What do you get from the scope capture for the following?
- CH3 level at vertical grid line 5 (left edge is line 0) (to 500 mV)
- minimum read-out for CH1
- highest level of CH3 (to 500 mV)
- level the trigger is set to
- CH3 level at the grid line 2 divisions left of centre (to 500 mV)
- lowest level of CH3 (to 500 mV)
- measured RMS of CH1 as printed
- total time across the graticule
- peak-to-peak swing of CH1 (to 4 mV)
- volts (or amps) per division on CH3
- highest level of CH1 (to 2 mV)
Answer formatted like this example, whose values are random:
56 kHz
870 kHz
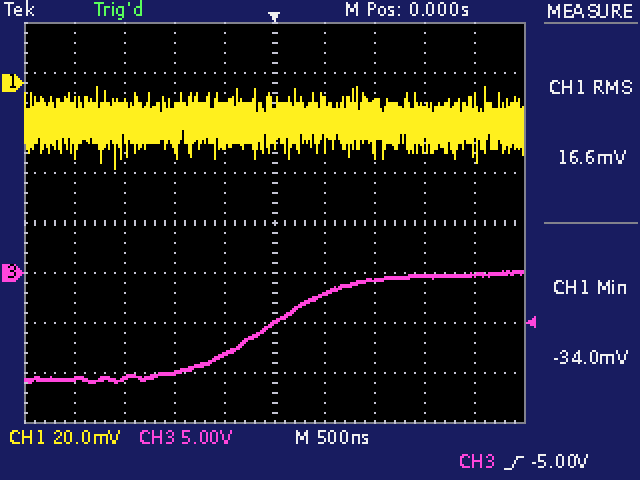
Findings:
-5.0 V
-34.0 mV
0.0 V
-5.00 V
-10.0 V
-11.0 V
16.6 mV
5 µs
32 mV
5 V
-2 mV
